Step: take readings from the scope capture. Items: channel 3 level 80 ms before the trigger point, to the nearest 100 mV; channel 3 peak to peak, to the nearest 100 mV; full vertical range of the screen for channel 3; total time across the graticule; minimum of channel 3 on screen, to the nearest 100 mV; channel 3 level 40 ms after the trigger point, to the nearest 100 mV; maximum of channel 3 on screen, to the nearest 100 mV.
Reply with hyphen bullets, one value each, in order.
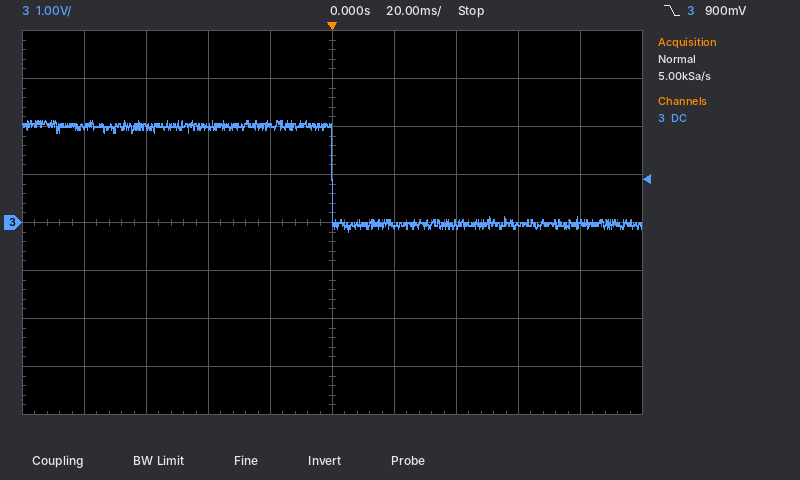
- 2.0 V
- 2.3 V
- 8 V
- 200 ms
- -200 mV
- 0.0 V
- 2.1 V
